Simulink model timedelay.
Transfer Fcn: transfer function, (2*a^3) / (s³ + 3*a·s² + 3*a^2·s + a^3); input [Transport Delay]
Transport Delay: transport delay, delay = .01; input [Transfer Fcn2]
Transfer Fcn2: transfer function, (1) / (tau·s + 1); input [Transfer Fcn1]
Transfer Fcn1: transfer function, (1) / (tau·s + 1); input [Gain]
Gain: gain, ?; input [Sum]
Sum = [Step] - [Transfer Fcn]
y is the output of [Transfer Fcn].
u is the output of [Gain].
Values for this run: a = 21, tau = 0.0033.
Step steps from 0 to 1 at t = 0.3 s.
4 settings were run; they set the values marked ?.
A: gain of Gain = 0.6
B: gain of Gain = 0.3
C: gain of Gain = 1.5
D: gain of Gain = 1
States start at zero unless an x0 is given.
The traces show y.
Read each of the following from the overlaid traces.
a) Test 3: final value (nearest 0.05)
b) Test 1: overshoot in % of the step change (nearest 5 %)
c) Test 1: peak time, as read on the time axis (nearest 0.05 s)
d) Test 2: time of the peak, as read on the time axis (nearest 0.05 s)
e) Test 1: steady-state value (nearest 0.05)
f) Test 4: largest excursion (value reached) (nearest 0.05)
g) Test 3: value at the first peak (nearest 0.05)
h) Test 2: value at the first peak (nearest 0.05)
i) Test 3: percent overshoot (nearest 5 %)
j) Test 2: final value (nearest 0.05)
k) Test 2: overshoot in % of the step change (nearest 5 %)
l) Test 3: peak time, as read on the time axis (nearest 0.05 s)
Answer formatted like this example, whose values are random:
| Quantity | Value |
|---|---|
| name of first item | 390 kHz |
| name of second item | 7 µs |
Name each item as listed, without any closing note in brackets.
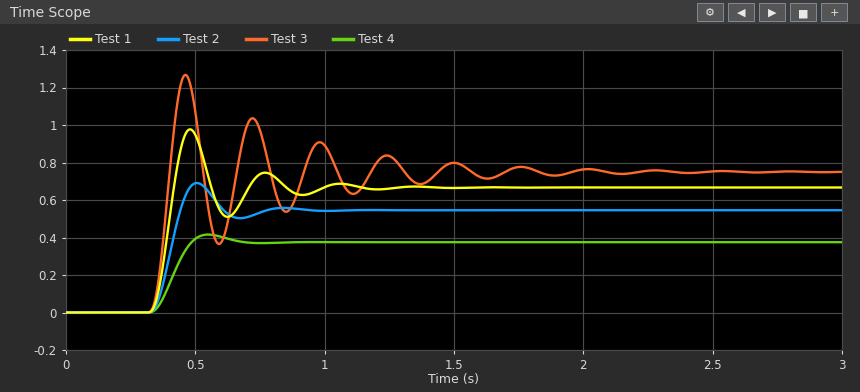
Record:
| Quantity | Value |
|---|---|
| Test 3: final value | 0.75 |
| Test 1: overshoot in % of the step change | 45 % |
| Test 1: peak time, as read on the time axis | 0.50 s |
| Test 2: time of the peak, as read on the time axis | 0.50 s |
| Test 1: steady-state value | 0.65 |
| Test 4: largest excursion (value reached) | 0.40 |
| Test 3: value at the first peak | 1.25 |
| Test 2: value at the first peak | 0.70 |
| Test 3: percent overshoot | 70 % |
| Test 2: final value | 0.55 |
| Test 2: overshoot in % of the step change | 25 % |
| Test 3: peak time, as read on the time axis | 0.45 s |
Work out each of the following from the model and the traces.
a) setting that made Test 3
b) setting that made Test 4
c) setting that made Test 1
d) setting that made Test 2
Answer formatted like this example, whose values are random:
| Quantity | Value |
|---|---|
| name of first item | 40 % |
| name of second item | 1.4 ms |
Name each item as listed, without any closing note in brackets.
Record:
| Quantity | Value |
|---|---|
| setting that made Test 3 | C |
| setting that made Test 4 | B |
| setting that made Test 1 | D |
| setting that made Test 2 | A |
